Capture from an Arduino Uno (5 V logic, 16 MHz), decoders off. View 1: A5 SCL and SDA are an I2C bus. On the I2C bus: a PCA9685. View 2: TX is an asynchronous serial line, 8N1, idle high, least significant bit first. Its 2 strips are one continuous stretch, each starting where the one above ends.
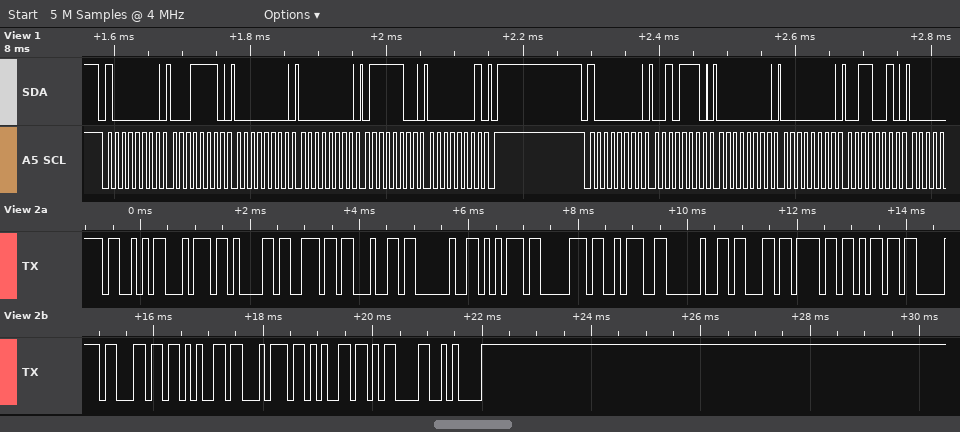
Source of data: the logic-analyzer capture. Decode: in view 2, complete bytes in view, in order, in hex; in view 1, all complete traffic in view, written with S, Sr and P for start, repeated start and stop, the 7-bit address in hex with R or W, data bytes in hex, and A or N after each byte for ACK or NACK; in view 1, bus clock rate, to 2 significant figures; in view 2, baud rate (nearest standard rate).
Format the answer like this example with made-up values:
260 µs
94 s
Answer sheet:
53 74 61 6E 64 20 75 70 3A 20 63 6F 6D 70 6C 65 74 65 0D 0A
S 40W A 1E A 00 A 00 A 7C A 01 A P S 40W A 2E A 00 A 00 A 32 A
100 kHz
9600 baud
